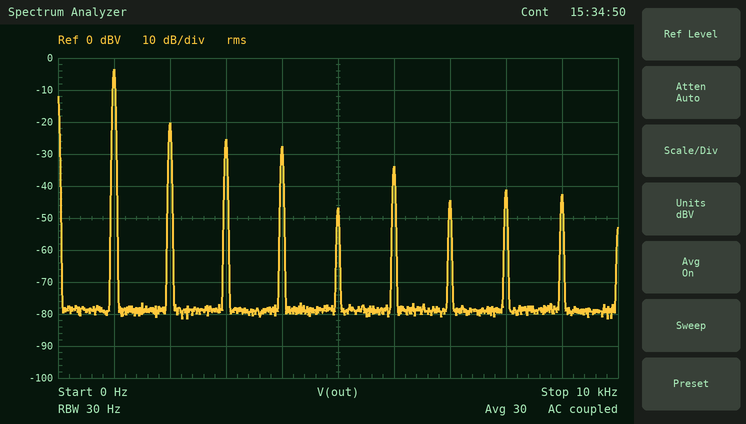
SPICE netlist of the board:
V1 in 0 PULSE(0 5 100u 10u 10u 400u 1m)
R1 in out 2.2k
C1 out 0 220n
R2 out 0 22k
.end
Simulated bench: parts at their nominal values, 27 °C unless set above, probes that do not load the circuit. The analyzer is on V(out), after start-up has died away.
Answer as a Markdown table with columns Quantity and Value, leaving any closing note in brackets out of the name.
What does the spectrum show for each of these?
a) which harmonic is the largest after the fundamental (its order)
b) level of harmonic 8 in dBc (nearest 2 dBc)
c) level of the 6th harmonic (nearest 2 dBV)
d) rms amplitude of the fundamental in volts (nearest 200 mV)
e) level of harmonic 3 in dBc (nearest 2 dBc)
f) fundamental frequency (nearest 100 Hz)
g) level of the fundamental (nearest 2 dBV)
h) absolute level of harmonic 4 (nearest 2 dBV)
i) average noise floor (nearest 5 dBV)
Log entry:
| Quantity | Value |
|---|---|
| which harmonic is the largest after the fundamental | 2 |
| level of harmonic 8 in dBc | -38 dBc |
| level of the 6th harmonic | -34 dBV |
| rms amplitude of the fundamental in volts | 600 mV |
| level of harmonic 3 in dBc | -22 dBc |
| fundamental frequency | 1.0 kHz |
| level of the fundamental | -4 dBV |
| absolute level of harmonic 4 | -28 dBV |
| average noise floor | -80 dBV |
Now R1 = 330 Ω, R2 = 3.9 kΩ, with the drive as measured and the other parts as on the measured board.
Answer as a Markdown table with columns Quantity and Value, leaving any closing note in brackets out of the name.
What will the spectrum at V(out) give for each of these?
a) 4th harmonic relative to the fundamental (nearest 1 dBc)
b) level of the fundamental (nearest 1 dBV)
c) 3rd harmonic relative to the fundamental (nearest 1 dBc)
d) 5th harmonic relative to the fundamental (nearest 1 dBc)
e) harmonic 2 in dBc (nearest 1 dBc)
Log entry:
| Quantity | Value |
|---|---|
| 4th harmonic relative to the fundamental | -18 dBc |
| level of the fundamental | 5 dBV |
| 3rd harmonic relative to the fundamental | -16 dBc |
| 5th harmonic relative to the fundamental | -36 dBc |
| harmonic 2 in dBc | -13 dBc |
